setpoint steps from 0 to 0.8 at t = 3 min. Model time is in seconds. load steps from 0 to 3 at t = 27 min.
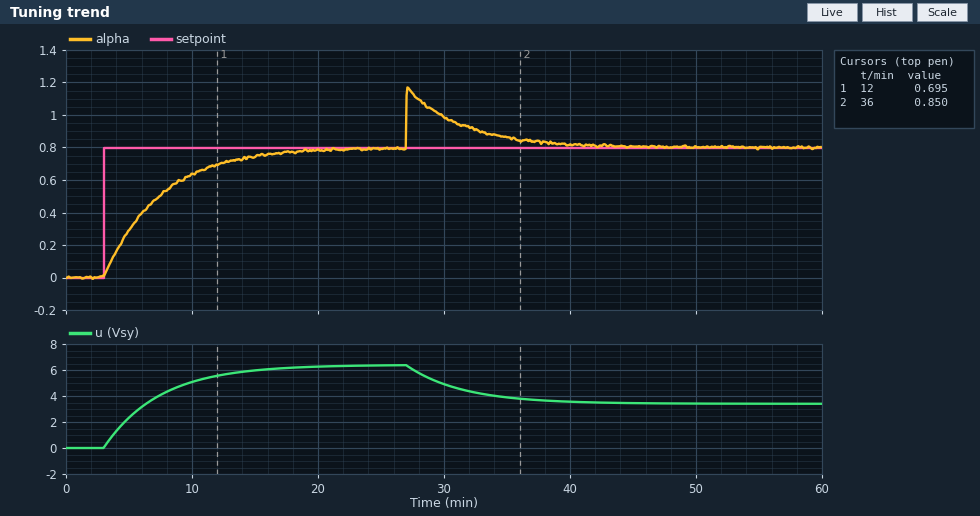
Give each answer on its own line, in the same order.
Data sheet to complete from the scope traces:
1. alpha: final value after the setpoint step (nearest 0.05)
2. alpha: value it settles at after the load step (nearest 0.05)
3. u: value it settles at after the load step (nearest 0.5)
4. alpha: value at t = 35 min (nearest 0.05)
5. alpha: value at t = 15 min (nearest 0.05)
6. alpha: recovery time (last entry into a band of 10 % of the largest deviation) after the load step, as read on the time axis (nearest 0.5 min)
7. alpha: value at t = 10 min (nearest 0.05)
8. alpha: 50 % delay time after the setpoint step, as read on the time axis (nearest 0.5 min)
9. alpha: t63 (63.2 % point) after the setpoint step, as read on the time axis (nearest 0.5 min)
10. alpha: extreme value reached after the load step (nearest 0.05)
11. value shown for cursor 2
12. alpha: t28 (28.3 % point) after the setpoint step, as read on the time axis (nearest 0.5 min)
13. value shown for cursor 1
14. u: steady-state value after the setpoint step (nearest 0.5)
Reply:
0.80
0.80
3.5
0.85
0.75
37.5 min
0.65
6.0 min
7.5 min
1.15
0.850
4.5 min
0.695
6.5
